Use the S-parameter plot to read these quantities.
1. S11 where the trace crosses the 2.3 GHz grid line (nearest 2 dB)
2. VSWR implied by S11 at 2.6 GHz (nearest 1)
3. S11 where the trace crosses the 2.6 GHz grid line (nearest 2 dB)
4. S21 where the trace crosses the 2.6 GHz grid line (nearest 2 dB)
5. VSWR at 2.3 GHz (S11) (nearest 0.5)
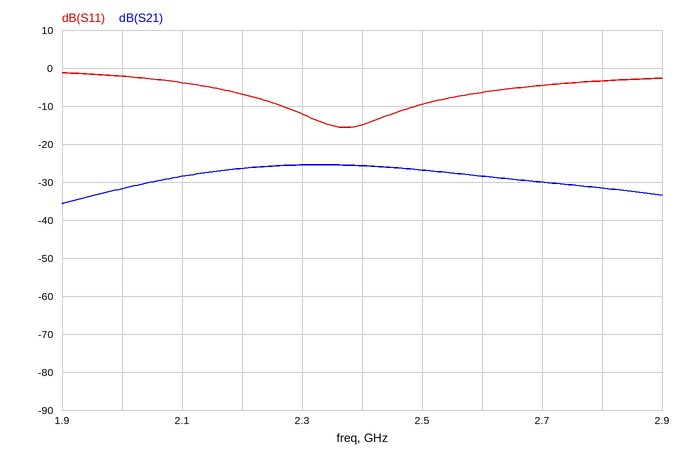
-12 dB
3
-6 dB
-28 dB
1.5
